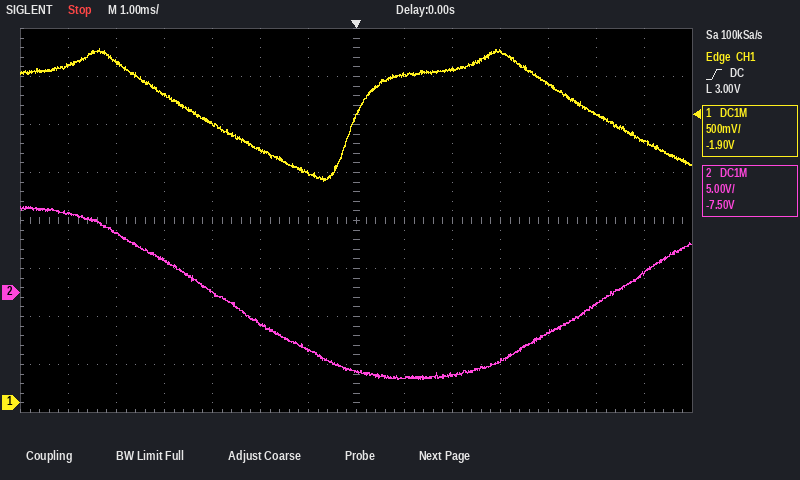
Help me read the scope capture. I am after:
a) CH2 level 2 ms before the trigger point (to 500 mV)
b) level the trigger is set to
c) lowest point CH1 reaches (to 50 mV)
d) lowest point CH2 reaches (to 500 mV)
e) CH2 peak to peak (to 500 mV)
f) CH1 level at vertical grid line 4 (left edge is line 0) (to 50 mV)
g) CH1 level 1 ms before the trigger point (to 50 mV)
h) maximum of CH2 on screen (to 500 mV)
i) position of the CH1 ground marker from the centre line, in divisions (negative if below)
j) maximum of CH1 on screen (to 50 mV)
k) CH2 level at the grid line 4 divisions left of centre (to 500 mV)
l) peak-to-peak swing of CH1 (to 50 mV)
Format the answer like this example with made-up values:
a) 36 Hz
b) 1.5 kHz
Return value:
a) -3.5 V
b) 3.00 V
c) 2.30 V
d) -9.0 V
e) 18.0 V
f) 2.90 V
g) 2.40 V
h) 9.0 V
i) -3.8 div
j) 3.70 V
k) 3.5 V
l) 1.40 V
